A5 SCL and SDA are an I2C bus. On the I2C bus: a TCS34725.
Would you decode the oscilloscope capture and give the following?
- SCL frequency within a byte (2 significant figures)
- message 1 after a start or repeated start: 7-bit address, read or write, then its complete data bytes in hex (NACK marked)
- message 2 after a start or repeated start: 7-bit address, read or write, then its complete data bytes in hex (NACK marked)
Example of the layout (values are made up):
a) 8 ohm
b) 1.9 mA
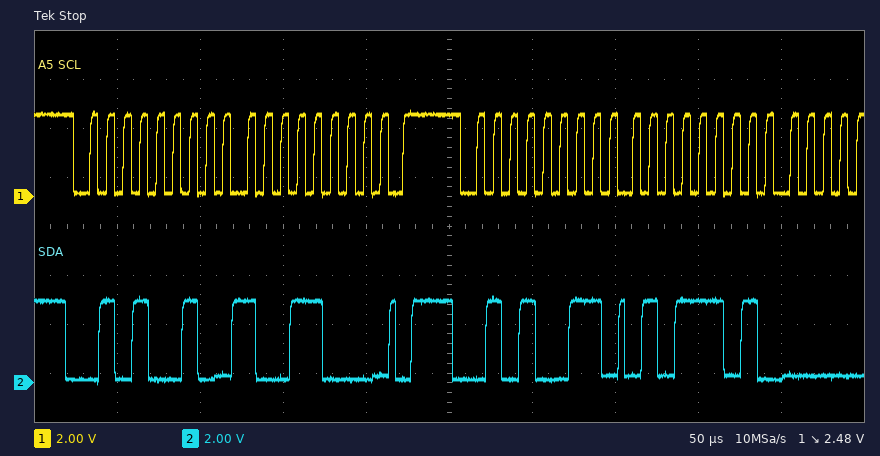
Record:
a) 100 kHz
b) 0x29 write: 98
c) 0x29 read: 5D
